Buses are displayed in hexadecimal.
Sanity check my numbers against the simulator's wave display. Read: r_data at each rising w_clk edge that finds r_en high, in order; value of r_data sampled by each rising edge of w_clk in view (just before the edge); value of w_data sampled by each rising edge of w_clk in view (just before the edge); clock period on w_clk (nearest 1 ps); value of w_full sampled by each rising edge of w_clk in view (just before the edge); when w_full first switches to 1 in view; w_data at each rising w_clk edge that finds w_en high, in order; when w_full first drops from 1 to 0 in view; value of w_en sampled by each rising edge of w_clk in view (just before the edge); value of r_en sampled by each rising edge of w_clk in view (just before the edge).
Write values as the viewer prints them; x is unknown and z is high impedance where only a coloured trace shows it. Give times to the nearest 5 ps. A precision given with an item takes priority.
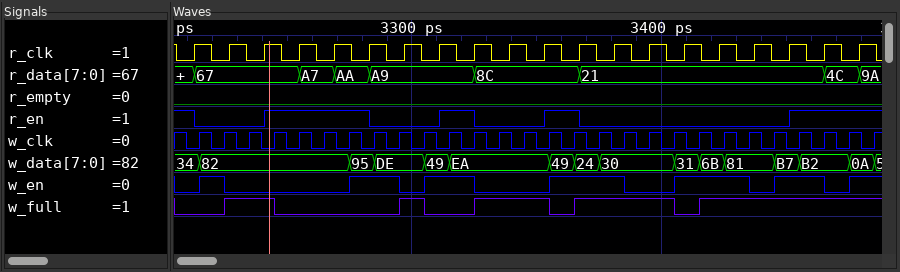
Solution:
67, 67, A7, AA, A9, A9, 8C, 8C, 21, 21, 4C, 9A
67, 67, 67, 67, 67, A7, AA, A9, A9, A9, A9, A9, 8C, 8C, 8C, 8C, 21, 21, 21, 21, 21, 21, 21, 21, 21, 21, 4C, 9A
34, 82, 82, 82, 82, 82, 82, 95, DE, DE, 49, EA, EA, EA, EA, 49, 24, 30, 30, 30, 31, 6B, 81, 81, B7, B2, B2, 0A
10 ps
0 0 1 1 0 0 0 0 0 1 0 0 1 1 1 0 1 1 1 1 0 1 1 1 1 1 1 1
3225 ps
82, 95, DE, 49, EA, 49, 24, 30, 31, 6B, 81, B7, B2, 0A
3245 ps
0 1 0 0 0 0 0 1 1 0 1 1 0 0 0 1 1 1 0 0 1 1 1 0 1 1 0 1
0 0 0 1 1 1 1 0 0 0 1 1 0 0 1 1 0 0 0 0 0 0 0 0 1 1 1 1
